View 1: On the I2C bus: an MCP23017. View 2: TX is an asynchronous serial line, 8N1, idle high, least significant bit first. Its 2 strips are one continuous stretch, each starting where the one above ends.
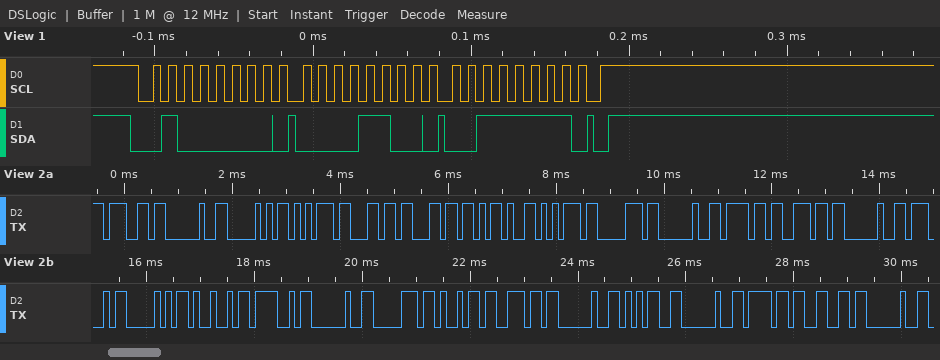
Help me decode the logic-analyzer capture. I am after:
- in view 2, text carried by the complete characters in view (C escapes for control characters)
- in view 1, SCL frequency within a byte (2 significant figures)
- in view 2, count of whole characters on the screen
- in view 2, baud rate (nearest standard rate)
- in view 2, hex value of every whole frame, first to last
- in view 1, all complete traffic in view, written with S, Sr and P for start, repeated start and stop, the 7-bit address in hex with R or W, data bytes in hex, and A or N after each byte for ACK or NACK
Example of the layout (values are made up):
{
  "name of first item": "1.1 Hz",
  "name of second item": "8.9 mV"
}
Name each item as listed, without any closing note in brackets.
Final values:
{
  "in view 2, text carried by the complete characters in view": "\"g Pull-up on GPIO pin 5 of \"",
  "in view 1, SCL frequency within a byte": "100 kHz",
  "in view 2, count of whole characters on the screen": "27",
  "in view 2, baud rate": "9600 baud",
  "in view 2, hex value of every whole frame, first to last": "67 20 50 75 6C 6C 2D 75 70 20 6F 6E 20 47 50 49 4F 20 70 69 6E 20 35 20 6F 66 20",
  "in view 1, all complete traffic in view, written with S, Sr and P for start, repeated start and stop, the 7-bit address in hex with R or W, data bytes in hex, and A or N after each byte for ACK or NACK": "S 20W A 0C A 3F A P"
}
